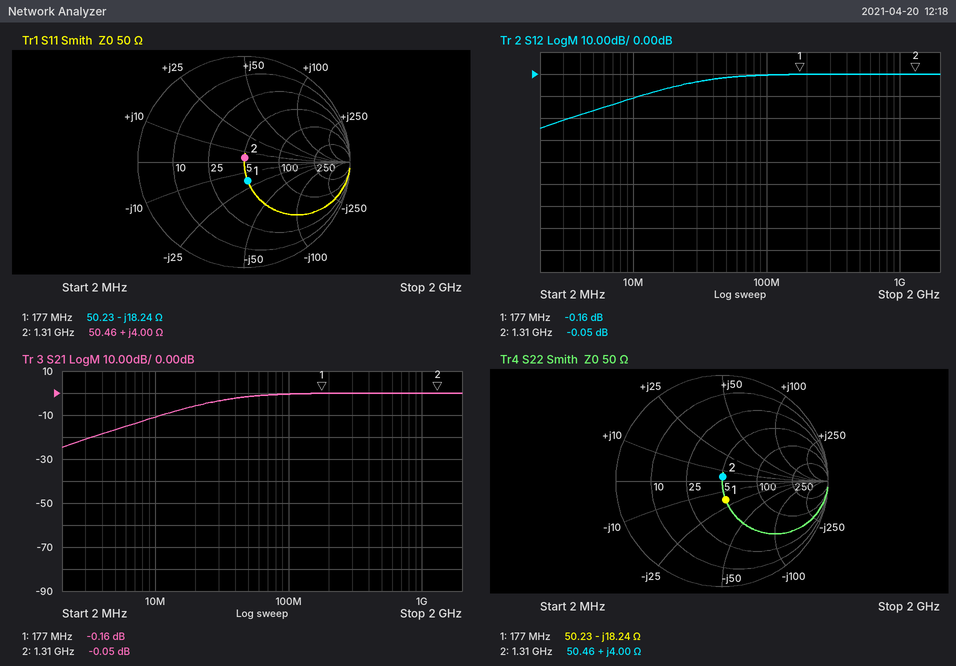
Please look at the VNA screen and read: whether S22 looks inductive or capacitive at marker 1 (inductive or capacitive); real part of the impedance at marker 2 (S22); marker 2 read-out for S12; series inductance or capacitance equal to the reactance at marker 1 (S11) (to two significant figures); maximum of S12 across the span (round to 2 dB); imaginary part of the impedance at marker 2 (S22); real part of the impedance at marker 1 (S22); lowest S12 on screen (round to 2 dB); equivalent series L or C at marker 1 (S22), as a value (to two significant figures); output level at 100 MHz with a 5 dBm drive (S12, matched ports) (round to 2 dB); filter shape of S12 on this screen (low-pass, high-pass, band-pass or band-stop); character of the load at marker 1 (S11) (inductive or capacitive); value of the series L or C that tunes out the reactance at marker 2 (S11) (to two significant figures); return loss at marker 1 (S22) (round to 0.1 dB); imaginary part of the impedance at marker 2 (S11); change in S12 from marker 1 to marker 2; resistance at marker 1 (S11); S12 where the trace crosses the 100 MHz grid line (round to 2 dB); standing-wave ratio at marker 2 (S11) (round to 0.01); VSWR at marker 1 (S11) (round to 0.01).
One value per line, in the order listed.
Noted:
capacitive
50.46 Ω
-0.05 dB
49 pF
0 dB
+4.00 Ω
50.23 Ω
-24 dB
49 pF
4 dBm
high-pass
capacitive
30 pF
14.9 dB
+4.00 Ω
0.11 dB
50.23 Ω
0 dB
1.08
1.44
